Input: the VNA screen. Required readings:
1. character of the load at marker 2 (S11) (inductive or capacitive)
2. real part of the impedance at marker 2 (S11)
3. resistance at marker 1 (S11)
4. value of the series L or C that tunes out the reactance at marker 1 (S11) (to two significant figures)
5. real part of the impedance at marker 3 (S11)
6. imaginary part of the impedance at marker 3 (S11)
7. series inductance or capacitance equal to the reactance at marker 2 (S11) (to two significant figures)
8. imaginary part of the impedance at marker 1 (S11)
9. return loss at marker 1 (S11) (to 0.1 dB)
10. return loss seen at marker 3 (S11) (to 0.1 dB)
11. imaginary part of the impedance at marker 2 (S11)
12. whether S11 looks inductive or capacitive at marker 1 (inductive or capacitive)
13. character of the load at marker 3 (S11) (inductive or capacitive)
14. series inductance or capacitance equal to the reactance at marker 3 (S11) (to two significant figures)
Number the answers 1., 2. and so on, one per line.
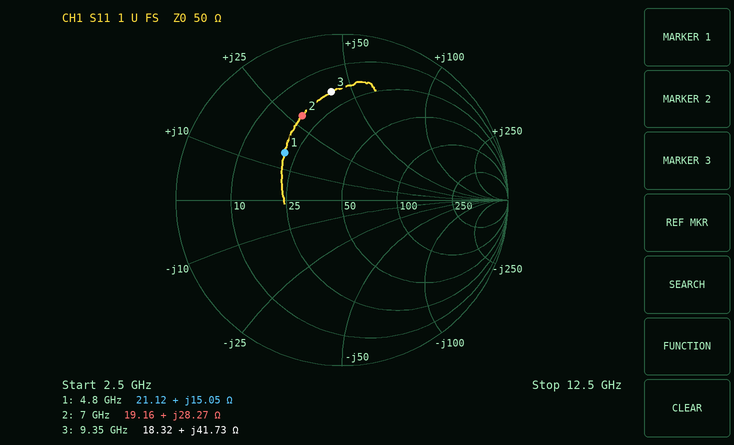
1. inductive
2. 19.16 Ω
3. 21.12 Ω
4. 2.2 pF
5. 18.32 Ω
6. +41.73 Ω
7. 640 pH
8. +15.05 Ω
9. 7.0 dB
10. 3.7 dB
11. +28.27 Ω
12. inductive
13. inductive
14. 710 pH
